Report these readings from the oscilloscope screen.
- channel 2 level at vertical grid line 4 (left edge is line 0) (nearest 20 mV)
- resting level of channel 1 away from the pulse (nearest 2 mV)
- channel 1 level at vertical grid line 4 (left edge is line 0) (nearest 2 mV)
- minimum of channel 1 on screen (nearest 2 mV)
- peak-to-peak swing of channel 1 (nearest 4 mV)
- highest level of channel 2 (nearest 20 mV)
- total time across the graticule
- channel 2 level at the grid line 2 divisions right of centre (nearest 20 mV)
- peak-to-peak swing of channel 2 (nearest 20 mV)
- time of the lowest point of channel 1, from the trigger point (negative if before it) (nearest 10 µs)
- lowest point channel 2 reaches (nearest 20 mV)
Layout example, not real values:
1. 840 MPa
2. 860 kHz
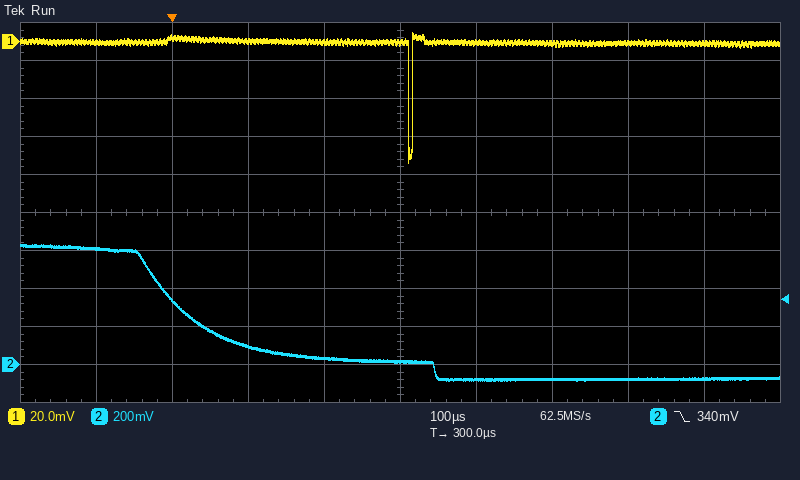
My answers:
1. 40 mV
2. 0 mV
3. 0 mV
4. -64 mV
5. 68 mV
6. 640 mV
7. 1 ms
8. -80 mV
9. 720 mV
10. +310 µs
11. -80 mV
